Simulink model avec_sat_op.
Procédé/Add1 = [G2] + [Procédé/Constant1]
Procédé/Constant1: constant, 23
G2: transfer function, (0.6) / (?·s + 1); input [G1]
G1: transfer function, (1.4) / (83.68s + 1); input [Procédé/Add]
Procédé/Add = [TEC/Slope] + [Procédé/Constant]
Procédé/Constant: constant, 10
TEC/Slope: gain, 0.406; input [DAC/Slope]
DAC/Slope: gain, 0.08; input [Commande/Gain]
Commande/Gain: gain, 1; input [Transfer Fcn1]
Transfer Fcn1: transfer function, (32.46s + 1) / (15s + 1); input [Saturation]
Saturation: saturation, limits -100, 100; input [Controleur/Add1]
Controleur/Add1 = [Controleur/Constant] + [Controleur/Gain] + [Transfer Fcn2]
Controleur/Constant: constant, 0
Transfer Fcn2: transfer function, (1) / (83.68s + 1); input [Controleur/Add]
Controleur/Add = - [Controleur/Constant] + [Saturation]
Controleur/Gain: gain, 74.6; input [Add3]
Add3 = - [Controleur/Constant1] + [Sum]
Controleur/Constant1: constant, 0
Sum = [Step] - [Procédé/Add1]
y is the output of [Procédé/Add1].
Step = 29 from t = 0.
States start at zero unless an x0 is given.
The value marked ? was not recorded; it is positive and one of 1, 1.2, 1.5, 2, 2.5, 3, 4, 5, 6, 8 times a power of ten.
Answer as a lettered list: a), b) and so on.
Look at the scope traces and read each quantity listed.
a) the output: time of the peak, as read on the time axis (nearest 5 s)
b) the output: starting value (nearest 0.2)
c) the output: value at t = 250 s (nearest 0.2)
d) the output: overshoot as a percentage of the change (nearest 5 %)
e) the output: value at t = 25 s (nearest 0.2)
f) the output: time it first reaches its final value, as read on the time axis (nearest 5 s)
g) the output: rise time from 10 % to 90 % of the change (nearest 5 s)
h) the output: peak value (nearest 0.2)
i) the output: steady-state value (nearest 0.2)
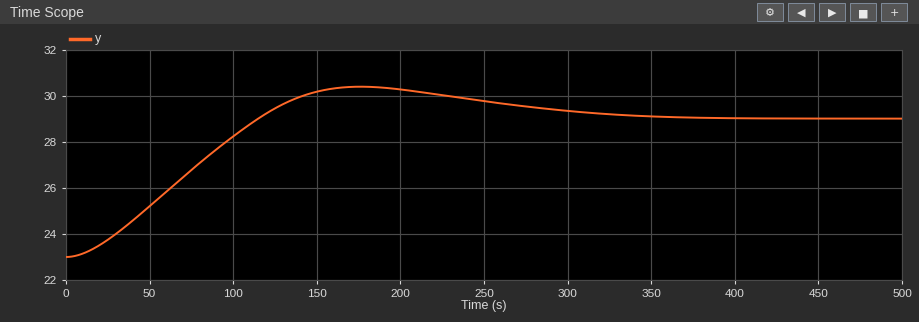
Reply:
a) 175 s
b) 23.0
c) 29.8
d) 25 %
e) 23.8
f) 115 s
g) 80 s
h) 30.4
i) 29.0
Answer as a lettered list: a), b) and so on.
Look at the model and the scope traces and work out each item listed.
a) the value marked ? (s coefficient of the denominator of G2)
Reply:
a) 50
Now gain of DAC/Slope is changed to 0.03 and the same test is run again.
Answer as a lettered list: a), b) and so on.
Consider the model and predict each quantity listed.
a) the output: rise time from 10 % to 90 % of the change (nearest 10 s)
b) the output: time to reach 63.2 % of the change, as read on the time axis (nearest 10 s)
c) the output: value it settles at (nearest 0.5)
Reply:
a) 130 s
b) 110 s
c) 30.5
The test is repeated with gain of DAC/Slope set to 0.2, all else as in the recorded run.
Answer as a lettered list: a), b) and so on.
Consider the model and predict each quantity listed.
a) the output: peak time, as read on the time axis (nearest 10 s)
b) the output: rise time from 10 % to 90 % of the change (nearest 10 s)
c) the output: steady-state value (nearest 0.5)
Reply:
a) 120 s
b) 60 s
c) 29.0
